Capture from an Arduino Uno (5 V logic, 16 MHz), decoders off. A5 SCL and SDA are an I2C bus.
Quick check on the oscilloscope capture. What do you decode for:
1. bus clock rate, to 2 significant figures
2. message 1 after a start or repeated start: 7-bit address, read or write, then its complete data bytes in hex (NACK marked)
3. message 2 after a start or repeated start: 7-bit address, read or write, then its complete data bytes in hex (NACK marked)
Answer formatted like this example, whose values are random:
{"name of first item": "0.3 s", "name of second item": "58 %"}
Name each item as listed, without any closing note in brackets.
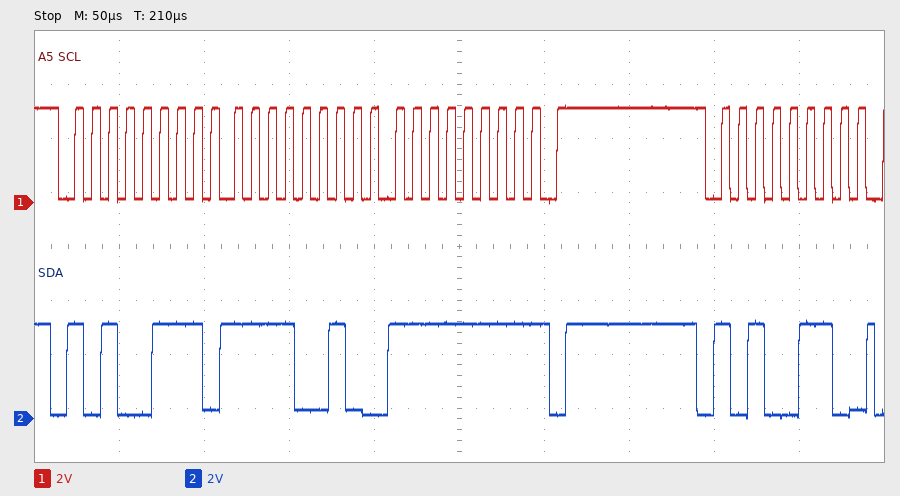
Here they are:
{"bus clock rate, to 2 significant figures": "100 kHz", "message 1 after a start or repeated start: 7-bit address, read or write, then its complete data bytes in hex": "0x53 read: F2 FF NACK", "message 2 after a start or repeated start: 7-bit address, read or write, then its complete data bytes in hex": "0x53 write"}
